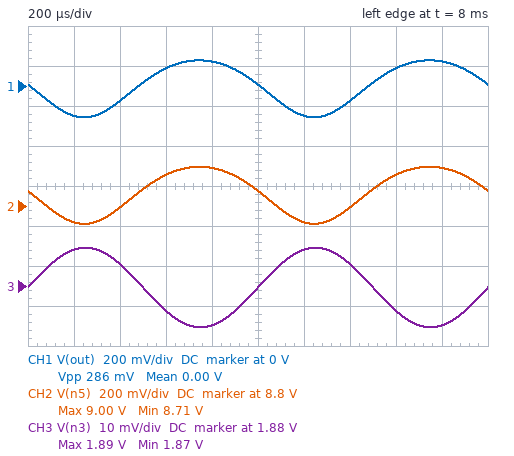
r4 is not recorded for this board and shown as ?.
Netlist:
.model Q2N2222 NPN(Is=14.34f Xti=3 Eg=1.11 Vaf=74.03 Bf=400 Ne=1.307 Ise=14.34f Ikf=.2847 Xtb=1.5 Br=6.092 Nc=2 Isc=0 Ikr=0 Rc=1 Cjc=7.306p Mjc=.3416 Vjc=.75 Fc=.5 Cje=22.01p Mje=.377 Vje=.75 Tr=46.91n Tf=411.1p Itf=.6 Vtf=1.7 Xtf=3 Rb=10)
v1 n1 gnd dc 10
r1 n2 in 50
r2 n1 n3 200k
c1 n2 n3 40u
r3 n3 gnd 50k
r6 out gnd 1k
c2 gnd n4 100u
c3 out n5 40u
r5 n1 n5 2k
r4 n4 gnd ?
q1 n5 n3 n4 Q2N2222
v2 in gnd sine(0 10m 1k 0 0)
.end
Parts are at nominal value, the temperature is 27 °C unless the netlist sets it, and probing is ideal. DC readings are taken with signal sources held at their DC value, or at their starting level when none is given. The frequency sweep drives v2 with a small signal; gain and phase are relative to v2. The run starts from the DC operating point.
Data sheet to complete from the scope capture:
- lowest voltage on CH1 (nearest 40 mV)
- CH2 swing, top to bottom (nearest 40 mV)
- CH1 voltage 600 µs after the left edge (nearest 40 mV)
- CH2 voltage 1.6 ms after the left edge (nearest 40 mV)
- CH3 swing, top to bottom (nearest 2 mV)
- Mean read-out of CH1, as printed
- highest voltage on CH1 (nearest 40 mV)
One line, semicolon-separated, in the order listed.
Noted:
-160 mV; 280 mV; 80 mV; 8.96 V; 20 mV; 0.00 V; 120 mV
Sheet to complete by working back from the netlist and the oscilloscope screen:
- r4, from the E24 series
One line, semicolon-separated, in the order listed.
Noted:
2.2 kΩ
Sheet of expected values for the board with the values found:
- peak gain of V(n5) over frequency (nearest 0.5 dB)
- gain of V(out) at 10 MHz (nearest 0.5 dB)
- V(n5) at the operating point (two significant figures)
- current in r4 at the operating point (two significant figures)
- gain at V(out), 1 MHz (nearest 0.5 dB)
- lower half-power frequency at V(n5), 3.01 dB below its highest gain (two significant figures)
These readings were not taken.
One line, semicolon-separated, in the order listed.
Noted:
23.0 dB; 22.5 dB; 8.9 V; 570 µA; 23.0 dB; 35 Hz
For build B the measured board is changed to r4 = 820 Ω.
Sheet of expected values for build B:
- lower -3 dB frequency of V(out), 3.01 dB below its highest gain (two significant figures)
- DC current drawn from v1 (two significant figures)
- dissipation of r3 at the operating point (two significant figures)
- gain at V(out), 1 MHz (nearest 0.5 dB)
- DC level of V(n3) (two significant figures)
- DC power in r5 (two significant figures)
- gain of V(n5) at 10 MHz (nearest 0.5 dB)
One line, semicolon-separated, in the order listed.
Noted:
82 Hz; 1.4 mA; 61 µW; 30.5 dB; 1.7 V; 3.5 mW; 28.5 dB
